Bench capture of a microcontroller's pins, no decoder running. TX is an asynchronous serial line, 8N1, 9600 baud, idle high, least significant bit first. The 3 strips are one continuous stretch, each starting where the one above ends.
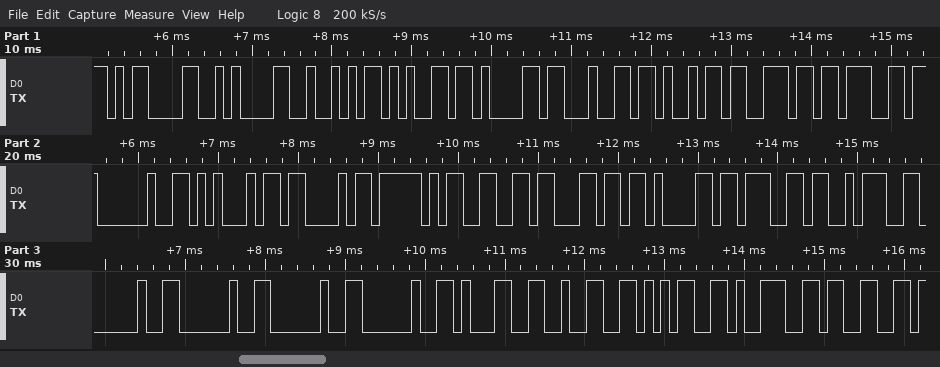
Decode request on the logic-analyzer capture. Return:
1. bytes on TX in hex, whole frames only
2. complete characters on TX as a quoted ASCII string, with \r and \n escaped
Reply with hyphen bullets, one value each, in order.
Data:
- 0D 0A 52 65 61 64 69 6E 67 20 45 43 5F 66 6C 61 67 3A 20 20 20 20 31 32 35 39 33
- "\r\nReading EC_flag:    12593"
